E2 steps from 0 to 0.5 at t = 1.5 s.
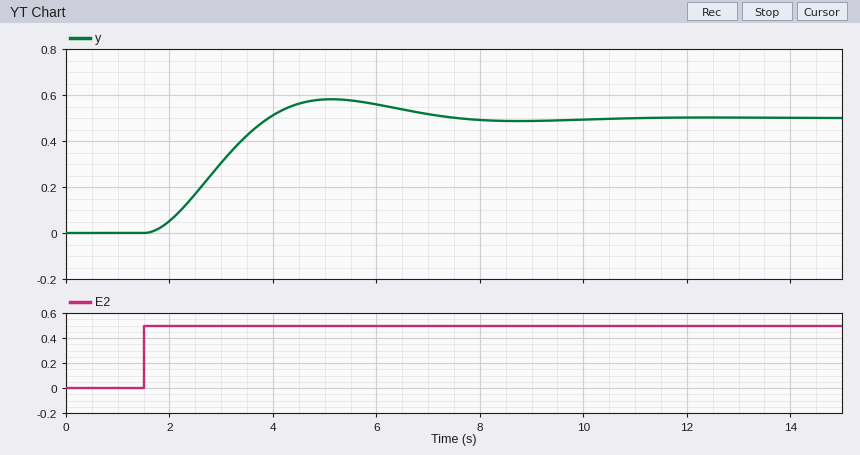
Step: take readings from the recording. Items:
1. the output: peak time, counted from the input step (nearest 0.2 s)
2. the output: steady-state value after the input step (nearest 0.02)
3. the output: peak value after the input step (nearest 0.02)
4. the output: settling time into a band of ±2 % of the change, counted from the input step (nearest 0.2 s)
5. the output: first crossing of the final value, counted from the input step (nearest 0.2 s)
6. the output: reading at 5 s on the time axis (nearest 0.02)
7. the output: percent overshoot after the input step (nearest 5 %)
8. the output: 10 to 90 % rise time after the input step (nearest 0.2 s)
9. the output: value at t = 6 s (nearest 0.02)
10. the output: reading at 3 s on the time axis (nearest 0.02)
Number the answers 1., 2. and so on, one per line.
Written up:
1. 3.6 s
2. 0.50
3. 0.58
4. 8.0 s
5. 2.4 s
6. 0.58
7. 15 %
8. 1.6 s
9. 0.56
10. 0.30
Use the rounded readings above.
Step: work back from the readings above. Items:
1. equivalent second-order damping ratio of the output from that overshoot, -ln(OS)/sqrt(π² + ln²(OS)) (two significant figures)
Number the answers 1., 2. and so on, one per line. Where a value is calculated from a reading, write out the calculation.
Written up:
1. ln(0.15) = -1.897; 1.897 / sqrt(9.870 + 3.599) = 0.52
